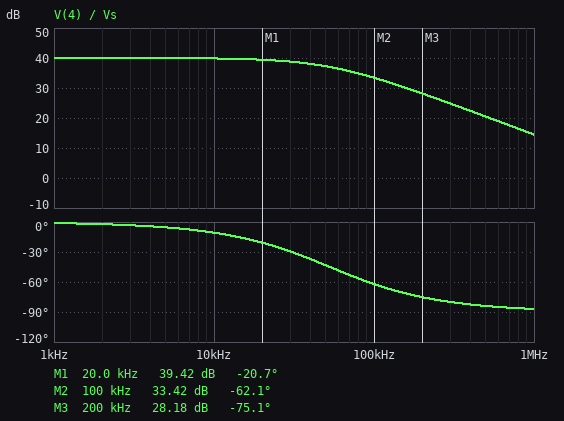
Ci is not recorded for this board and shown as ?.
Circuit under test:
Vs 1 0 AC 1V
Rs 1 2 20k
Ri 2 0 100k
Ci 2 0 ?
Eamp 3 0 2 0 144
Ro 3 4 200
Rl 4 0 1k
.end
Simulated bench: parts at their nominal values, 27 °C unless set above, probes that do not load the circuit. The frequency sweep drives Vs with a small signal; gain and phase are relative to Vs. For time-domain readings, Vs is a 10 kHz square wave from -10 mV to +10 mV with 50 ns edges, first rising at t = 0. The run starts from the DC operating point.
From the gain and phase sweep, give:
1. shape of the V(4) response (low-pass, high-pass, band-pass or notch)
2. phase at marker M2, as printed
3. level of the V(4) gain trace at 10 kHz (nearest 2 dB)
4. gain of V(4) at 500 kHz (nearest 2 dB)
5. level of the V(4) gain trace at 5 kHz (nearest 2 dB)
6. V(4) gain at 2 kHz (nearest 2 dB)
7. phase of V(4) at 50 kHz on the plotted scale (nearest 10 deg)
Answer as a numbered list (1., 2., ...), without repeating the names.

1. low-pass
2. -62.1 deg
3. 40 dB
4. 20 dB
5. 40 dB
6. 40 dB
7. -40 deg
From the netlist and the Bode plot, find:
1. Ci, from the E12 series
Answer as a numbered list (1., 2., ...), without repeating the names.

1. 180 pF
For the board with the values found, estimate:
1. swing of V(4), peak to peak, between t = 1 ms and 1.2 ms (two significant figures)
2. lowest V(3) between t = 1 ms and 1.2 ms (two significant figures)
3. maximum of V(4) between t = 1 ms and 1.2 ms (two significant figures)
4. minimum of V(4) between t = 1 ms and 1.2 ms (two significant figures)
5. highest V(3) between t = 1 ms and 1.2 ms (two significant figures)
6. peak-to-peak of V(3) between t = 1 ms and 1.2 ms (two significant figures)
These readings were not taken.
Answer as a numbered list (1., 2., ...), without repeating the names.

1. 2.0 V
2. -1.2 V
3. 1.0 V
4. -1.0 V
5. 1.2 V
6. 2.4 V
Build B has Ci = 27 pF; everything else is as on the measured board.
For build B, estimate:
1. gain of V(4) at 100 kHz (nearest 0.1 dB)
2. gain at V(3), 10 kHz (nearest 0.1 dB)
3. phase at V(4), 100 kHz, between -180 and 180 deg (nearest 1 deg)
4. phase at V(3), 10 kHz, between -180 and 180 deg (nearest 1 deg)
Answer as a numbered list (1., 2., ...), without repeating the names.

1. 39.7 dB
2. 41.6 dB
3. -16 deg
4. -2 deg
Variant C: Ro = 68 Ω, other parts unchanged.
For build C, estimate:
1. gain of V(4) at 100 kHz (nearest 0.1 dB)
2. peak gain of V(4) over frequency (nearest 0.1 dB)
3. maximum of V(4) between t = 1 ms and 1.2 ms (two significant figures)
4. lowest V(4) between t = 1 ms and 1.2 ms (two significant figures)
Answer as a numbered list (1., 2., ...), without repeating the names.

1. 34.4 dB
2. 41.0 dB
3. 1.1 V
4. -1.1 V
